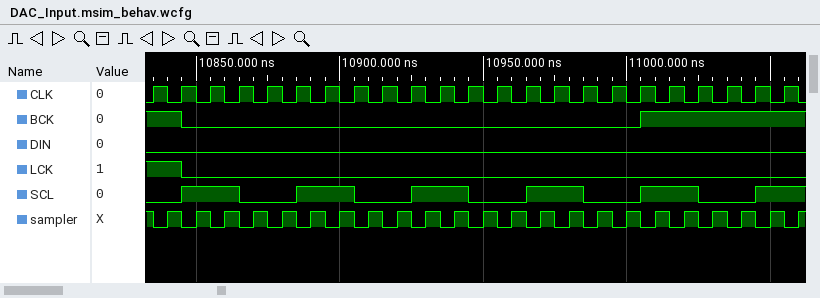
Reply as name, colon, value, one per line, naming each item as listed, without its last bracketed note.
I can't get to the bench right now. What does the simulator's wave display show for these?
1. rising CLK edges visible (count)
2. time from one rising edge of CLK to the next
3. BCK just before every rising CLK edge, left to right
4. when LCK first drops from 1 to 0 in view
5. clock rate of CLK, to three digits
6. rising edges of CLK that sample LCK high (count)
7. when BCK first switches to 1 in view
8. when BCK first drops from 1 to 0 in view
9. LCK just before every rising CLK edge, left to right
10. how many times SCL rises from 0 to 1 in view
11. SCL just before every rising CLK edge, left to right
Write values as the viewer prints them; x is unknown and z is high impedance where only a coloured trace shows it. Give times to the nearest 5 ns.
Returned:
rising CLK edges visible: 23
time from one rising edge of CLK to the next: 10 ns
BCK just before every rising CLK edge, left to right: 1 1 0 0 0 0 0 0 0 0 0 0 0 0 0 0 0 0 1 1 1 1 1
when LCK first drops from 1 to 0 in view: 10845 ns
clock rate of CLK, to three digits: 100 MHz
rising edges of CLK that sample LCK high: 2
when BCK first switches to 1 in view: 11005 ns
when BCK first drops from 1 to 0 in view: 10845 ns
LCK just before every rising CLK edge, left to right: 1 1 0 0 0 0 0 0 0 0 0 0 0 0 0 0 0 0 0 0 0 0 0
how many times SCL rises from 0 to 1 in view: 6
SCL just before every rising CLK edge, left to right: 0 0 1 1 0 0 1 1 0 0 1 1 0 0 1 1 0 0 1 1 0 0 1
